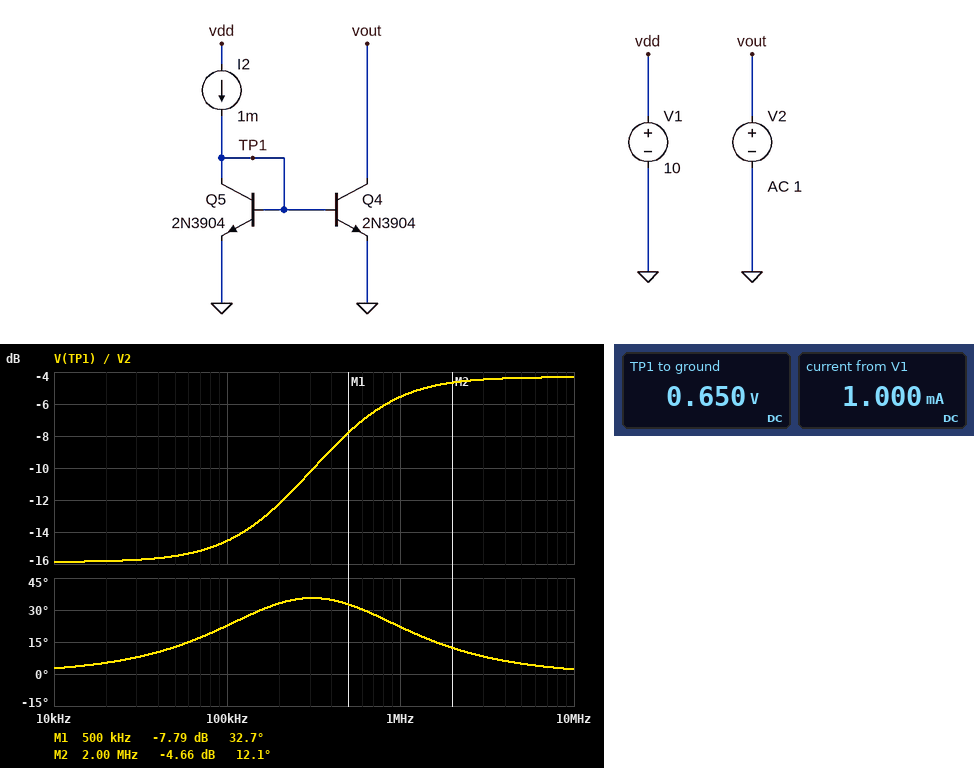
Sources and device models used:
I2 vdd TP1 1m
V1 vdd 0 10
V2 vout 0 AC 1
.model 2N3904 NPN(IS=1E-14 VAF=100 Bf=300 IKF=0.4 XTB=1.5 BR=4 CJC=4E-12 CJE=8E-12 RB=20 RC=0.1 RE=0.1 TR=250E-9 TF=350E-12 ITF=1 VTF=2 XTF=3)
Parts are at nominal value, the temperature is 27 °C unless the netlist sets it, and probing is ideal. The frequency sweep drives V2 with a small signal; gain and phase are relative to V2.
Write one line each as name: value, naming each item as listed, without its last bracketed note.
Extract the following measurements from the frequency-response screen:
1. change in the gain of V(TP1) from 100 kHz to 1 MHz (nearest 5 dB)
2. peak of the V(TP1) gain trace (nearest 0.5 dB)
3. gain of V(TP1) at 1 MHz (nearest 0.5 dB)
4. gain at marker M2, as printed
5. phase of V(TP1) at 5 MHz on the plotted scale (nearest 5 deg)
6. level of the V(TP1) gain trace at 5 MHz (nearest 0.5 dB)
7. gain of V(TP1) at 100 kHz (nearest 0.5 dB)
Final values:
change in the gain of V(TP1) from 100 kHz to 1 MHz: 10 dB
peak of the V(TP1) gain trace: -4.5 dB
gain of V(TP1) at 1 MHz: -5.5 dB
gain at marker M2, as printed: -4.66 dB
phase of V(TP1) at 5 MHz on the plotted scale: 5 deg
level of the V(TP1) gain trace at 5 MHz: -4.5 dB
gain of V(TP1) at 100 kHz: -14.5 dB
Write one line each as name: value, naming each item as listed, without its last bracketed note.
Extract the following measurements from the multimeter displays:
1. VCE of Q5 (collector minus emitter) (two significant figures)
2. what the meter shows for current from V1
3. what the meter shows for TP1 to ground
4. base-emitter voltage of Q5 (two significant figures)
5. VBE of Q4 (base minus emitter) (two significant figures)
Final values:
VCE of Q5 (collector minus emitter): 650 mV
what the meter shows for current from V1: 1.000 mA
what the meter shows for TP1 to ground: 0.650 V
base-emitter voltage of Q5: 650 mV
VBE of Q4 (base minus emitter): 650 mV
